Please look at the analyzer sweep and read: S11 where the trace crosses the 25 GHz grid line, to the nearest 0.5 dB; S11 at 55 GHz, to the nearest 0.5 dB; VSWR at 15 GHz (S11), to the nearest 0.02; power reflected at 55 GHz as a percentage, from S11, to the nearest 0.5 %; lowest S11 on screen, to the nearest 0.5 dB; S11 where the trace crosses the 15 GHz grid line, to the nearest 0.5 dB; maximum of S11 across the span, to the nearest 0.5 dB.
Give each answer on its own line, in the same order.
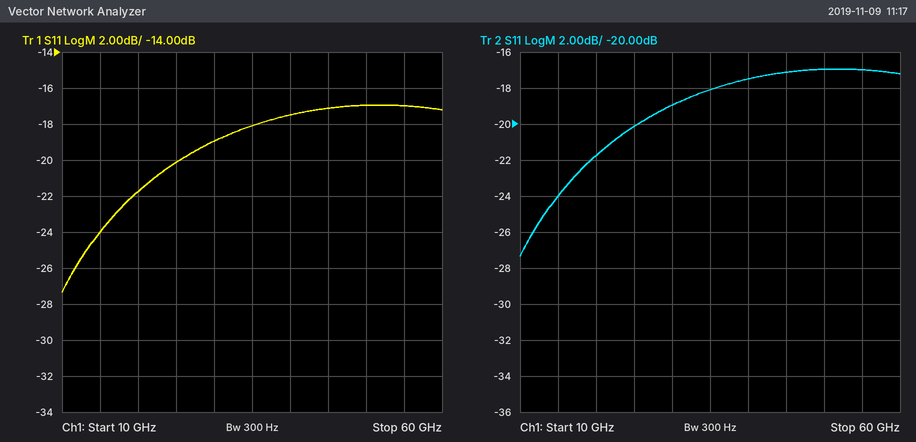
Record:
-20.0 dB
-17.0 dB
1.14
2.0 %
-27.5 dB
-24.0 dB
-17.0 dB
